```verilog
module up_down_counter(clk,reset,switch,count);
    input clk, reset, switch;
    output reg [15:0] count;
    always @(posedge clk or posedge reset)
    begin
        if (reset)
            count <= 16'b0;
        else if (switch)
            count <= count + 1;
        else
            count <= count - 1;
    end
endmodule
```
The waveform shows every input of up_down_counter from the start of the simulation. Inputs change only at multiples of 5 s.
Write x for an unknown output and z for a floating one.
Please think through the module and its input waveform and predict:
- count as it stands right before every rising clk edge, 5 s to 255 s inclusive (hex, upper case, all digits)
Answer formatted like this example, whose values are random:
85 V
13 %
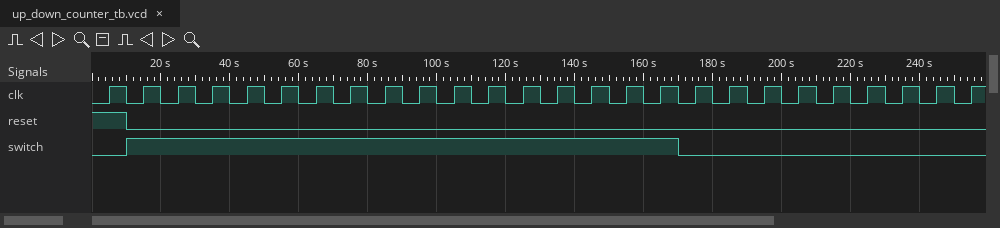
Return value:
0000, 0000, 0001, 0002, 0003, 0004, 0005, 0006, 0007, 0008, 0009, 000A, 000B, 000C, 000D, 000E, 000F, 0010, 000F, 000E, 000D, 000C, 000B, 000A, 0009, 0008
